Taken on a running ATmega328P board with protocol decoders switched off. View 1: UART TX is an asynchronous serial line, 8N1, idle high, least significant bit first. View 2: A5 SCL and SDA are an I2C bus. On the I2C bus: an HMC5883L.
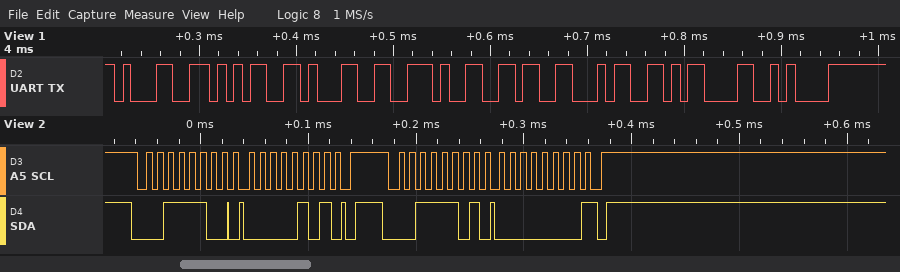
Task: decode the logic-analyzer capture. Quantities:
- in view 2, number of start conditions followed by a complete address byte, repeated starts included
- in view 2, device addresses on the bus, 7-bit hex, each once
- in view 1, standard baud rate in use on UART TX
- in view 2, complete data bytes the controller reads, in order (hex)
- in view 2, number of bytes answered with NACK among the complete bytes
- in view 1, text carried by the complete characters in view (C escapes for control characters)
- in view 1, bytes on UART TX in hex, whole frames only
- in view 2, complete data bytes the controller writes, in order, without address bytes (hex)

2
0x1E
115200 baud
00
1
"151.64\r\n"
31 35 31 2E 36 34 0D 0A
05
